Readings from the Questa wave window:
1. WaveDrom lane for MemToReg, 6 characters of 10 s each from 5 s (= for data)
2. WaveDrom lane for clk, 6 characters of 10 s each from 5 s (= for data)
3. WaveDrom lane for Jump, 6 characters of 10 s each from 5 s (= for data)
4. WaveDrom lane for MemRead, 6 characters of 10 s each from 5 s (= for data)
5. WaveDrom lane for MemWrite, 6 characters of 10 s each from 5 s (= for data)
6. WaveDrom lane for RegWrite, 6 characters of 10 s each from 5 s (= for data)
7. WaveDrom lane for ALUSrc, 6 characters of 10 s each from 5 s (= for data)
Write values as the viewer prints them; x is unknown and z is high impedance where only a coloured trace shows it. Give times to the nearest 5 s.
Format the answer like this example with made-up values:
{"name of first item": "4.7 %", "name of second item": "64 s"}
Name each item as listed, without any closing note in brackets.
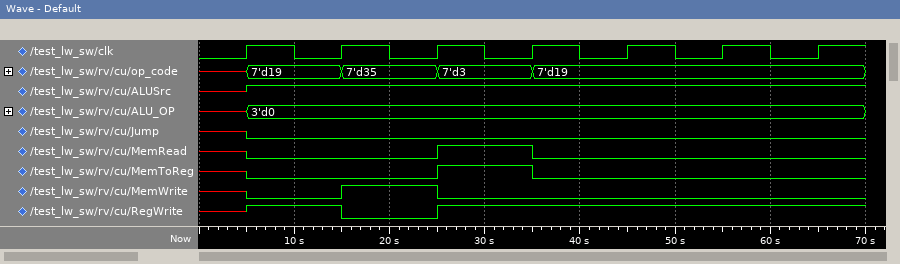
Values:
{"WaveDrom lane for MemToReg, 6 characters of 10 s each from 5 s": "{name: 'MemToReg', wave: '0.10..'}", "WaveDrom lane for clk, 6 characters of 10 s each from 5 s": "{name: 'clk', wave: 'p.....'}", "WaveDrom lane for Jump, 6 characters of 10 s each from 5 s": "{name: 'Jump', wave: '0.....'}", "WaveDrom lane for MemRead, 6 characters of 10 s each from 5 s": "{name: 'MemRead', wave: '0.10..'}", "WaveDrom lane for MemWrite, 6 characters of 10 s each from 5 s": "{name: 'MemWrite', wave: '010...'}", "WaveDrom lane for RegWrite, 6 characters of 10 s each from 5 s": "{name: 'RegWrite', wave: '101...'}", "WaveDrom lane for ALUSrc, 6 characters of 10 s each from 5 s": "{name: 'ALUSrc', wave: '1.....'}"}
